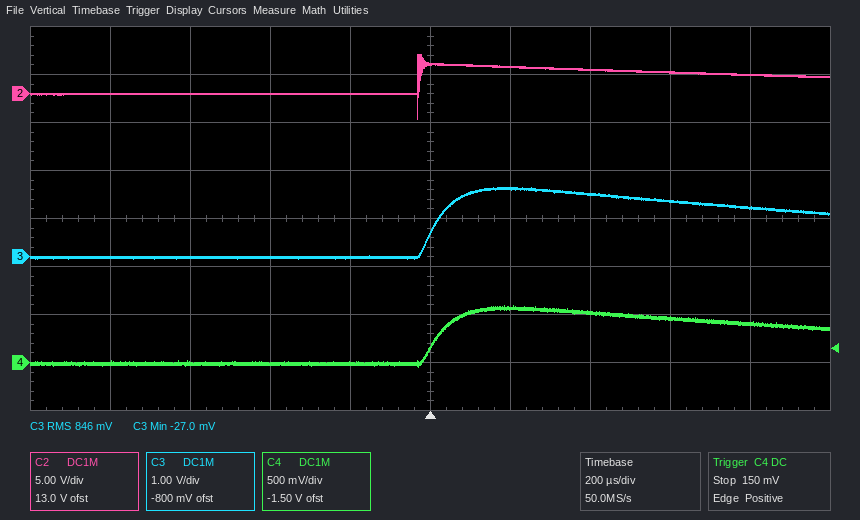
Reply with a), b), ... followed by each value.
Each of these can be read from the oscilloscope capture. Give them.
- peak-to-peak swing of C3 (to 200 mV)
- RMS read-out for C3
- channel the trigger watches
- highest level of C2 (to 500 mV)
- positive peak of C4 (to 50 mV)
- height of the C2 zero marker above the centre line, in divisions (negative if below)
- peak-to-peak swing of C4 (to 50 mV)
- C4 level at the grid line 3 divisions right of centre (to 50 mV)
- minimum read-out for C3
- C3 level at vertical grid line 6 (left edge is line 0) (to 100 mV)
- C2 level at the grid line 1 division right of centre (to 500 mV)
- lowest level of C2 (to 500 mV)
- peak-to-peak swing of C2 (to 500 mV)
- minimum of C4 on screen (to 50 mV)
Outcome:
a) 1.4 V
b) 846 mV
c) C4
d) 4.0 V
e) 600 mV
f) +2.6 div
g) 650 mV
h) 450 mV
i) -27.0 mV
j) 1.4 V
k) 3.0 V
l) -2.5 V
m) 6.5 V
n) -50 mV
